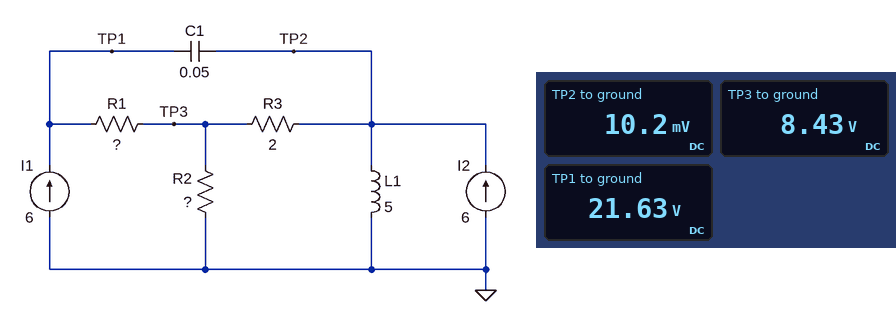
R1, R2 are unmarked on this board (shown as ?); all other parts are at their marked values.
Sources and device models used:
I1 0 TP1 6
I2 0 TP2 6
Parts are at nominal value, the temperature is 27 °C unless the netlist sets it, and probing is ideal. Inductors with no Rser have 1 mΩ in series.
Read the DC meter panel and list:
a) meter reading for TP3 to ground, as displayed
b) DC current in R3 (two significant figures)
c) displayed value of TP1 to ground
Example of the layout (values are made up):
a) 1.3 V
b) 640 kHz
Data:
a) 8.43 V
b) 4.2 A
c) 21.63 V
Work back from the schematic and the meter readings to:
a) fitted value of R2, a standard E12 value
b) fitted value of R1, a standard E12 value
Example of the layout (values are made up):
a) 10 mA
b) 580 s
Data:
a) 4.7 Ω
b) 2.2 Ω
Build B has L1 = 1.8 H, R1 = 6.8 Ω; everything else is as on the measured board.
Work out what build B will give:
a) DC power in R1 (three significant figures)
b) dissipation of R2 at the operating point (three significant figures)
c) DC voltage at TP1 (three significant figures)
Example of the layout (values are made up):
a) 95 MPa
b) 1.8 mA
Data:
a) 245 W
b) 15.1 W
c) 49.2 V
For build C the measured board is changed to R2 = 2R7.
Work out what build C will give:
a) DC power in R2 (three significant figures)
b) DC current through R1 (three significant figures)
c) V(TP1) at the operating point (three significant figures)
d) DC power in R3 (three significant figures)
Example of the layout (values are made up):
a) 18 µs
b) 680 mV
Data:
a) 17.6 W
b) 6.00 A
c) 20.1 V
d) 23.7 W
